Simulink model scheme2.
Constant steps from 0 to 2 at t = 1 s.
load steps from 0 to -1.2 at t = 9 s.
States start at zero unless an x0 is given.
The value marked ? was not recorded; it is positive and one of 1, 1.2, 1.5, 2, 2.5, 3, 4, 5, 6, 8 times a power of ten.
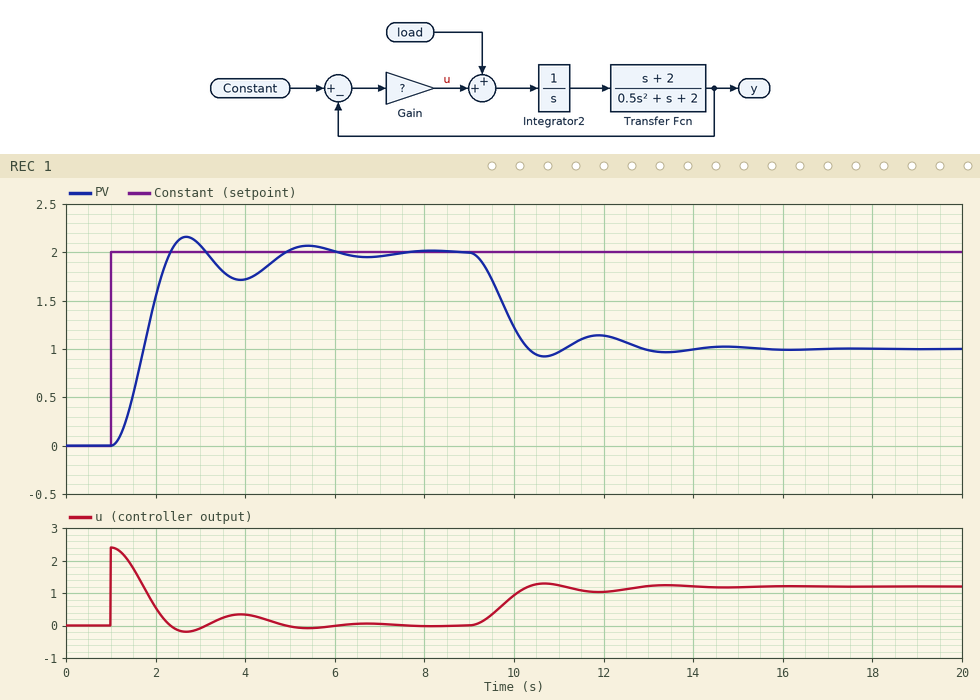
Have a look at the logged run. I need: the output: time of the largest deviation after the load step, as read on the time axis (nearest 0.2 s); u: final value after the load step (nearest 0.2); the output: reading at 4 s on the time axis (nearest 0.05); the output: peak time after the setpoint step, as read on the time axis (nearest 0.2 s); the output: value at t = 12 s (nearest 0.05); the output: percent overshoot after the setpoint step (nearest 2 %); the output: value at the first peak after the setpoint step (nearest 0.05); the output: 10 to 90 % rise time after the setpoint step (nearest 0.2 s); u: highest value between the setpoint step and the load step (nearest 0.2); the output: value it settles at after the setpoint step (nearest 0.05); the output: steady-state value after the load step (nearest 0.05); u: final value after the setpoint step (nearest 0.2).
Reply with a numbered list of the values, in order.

1. 10.6 s
2. 1.2
3. 1.70
4. 2.6 s
5. 1.15
6. 8 %
7. 2.15
8. 0.8 s
9. 2.4
10. 2.00
11. 1.00
12. 0.0
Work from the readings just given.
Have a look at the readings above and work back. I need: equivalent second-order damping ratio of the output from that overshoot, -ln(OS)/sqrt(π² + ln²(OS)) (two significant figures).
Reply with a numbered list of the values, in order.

1. 0.63
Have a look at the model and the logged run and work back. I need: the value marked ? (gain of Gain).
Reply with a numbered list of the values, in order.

1. 1.2
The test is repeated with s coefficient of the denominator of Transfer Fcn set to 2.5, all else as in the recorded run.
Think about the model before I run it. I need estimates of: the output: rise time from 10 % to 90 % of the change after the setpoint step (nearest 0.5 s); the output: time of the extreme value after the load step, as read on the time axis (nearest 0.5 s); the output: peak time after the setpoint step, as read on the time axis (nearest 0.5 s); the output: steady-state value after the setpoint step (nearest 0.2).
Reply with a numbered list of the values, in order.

1. 1.5 s
2. 12.0 s
3. 4.0 s
4. 2.0
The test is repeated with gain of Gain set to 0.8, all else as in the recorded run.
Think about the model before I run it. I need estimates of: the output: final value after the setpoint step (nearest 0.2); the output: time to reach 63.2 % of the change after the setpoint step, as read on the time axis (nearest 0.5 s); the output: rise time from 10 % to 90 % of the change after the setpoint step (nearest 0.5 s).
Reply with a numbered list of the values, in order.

1. 2.0
2. 2.0 s
3. 1.5 s
